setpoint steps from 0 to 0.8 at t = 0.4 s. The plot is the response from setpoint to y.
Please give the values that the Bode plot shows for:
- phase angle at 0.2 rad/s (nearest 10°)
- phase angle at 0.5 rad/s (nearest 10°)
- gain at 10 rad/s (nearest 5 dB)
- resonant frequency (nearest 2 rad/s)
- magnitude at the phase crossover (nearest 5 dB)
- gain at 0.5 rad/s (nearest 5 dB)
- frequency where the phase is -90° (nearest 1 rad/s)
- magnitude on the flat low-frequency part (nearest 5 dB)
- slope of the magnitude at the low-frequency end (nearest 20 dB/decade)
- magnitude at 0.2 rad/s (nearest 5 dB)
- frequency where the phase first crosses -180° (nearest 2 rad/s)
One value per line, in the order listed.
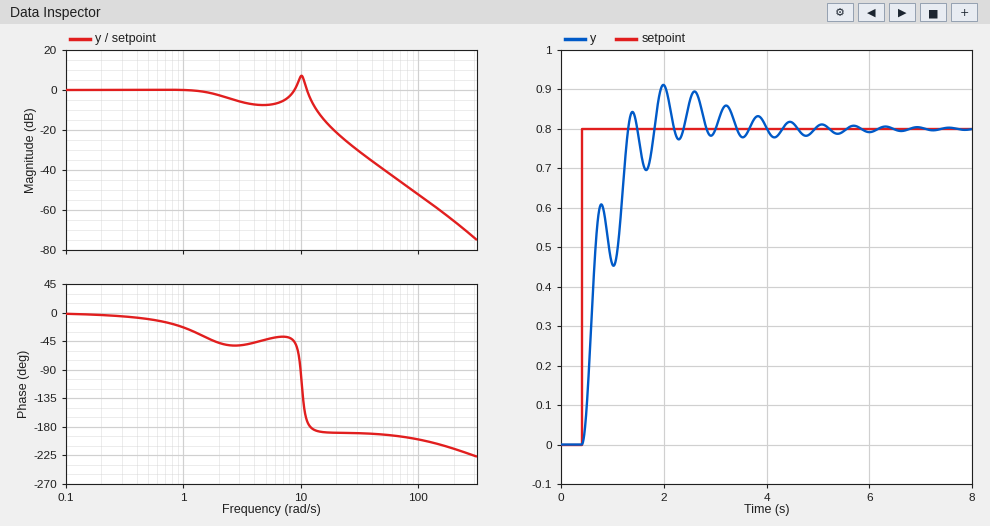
0°
-10°
5 dB
10 rad/s
-5 dB
0 dB
10 rad/s
0 dB
0 dB/decade
0 dB
12 rad/s
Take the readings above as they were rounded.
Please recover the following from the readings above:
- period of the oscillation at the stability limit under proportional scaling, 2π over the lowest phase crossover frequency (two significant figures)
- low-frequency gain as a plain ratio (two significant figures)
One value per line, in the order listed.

0.52 s
1.0
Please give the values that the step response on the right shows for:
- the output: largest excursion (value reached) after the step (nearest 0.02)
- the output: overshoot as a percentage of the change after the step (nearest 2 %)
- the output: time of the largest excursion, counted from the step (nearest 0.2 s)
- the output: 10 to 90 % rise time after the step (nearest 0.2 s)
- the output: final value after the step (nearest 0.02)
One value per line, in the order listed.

0.92
14 %
1.6 s
0.8 s
0.80
